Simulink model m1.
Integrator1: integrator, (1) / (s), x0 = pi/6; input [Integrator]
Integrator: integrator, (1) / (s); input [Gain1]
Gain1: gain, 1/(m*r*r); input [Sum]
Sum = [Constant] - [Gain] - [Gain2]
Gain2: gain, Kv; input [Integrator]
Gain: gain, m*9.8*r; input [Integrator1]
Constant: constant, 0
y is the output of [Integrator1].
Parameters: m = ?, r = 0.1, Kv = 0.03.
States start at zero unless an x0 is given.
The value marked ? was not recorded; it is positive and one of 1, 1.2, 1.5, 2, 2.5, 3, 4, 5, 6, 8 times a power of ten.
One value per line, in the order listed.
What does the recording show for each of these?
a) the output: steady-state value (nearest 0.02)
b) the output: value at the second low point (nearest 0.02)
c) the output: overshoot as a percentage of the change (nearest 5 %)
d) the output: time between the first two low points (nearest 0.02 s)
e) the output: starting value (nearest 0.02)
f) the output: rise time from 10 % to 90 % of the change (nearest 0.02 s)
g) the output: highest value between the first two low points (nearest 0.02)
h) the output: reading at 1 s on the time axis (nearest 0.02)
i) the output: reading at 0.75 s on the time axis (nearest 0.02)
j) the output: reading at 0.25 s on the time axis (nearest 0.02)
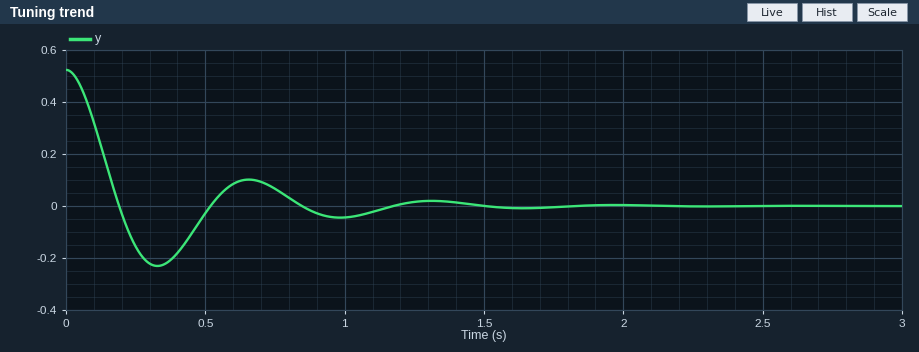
0.00
-0.04
45 %
0.66 s
0.52
0.12 s
0.10
-0.04
0.06
-0.16
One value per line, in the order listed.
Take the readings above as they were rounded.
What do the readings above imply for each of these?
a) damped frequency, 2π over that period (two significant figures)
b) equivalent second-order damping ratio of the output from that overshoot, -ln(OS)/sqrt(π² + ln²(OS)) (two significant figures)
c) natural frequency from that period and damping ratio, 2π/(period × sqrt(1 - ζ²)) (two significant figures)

9.5 rad/s
0.25
9.8 rad/s
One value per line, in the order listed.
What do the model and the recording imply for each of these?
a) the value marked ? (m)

0.6
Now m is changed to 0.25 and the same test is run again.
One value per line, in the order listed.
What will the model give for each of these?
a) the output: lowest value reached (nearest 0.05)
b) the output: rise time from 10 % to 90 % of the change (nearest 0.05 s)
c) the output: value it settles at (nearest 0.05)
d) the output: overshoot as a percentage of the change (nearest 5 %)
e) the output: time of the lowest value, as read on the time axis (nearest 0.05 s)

-0.05
0.20 s
0.00
10 %
0.40 s
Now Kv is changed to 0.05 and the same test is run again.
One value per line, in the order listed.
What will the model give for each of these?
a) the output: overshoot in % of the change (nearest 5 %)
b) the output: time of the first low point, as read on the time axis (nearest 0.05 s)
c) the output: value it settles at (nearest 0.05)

25 %
0.35 s
0.00
